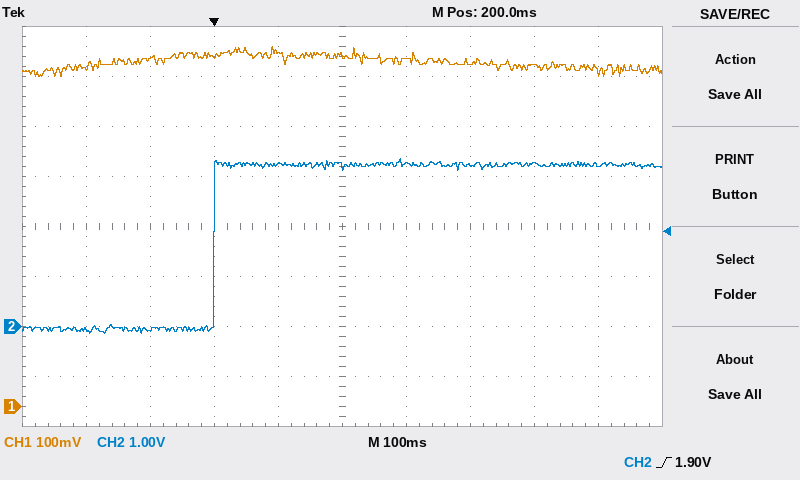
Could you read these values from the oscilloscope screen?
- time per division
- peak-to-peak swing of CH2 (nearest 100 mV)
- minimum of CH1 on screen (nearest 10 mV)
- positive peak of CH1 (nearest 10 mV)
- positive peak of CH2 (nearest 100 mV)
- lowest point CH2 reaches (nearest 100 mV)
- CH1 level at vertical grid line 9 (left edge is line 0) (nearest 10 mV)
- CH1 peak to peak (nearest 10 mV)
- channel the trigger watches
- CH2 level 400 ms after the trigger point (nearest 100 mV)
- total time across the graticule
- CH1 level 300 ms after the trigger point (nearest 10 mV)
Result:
100 ms
3.5 V
660 mV
720 mV
3.4 V
-100 mV
670 mV
60 mV
CH2
3.2 V
1 s
700 mV
